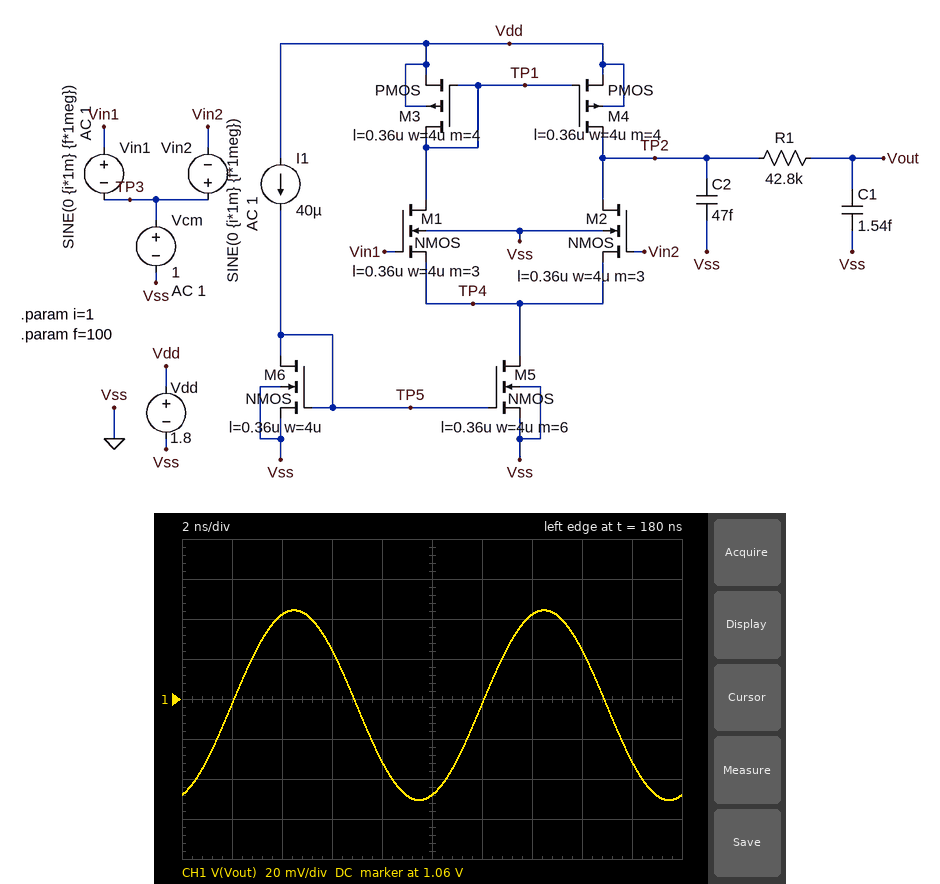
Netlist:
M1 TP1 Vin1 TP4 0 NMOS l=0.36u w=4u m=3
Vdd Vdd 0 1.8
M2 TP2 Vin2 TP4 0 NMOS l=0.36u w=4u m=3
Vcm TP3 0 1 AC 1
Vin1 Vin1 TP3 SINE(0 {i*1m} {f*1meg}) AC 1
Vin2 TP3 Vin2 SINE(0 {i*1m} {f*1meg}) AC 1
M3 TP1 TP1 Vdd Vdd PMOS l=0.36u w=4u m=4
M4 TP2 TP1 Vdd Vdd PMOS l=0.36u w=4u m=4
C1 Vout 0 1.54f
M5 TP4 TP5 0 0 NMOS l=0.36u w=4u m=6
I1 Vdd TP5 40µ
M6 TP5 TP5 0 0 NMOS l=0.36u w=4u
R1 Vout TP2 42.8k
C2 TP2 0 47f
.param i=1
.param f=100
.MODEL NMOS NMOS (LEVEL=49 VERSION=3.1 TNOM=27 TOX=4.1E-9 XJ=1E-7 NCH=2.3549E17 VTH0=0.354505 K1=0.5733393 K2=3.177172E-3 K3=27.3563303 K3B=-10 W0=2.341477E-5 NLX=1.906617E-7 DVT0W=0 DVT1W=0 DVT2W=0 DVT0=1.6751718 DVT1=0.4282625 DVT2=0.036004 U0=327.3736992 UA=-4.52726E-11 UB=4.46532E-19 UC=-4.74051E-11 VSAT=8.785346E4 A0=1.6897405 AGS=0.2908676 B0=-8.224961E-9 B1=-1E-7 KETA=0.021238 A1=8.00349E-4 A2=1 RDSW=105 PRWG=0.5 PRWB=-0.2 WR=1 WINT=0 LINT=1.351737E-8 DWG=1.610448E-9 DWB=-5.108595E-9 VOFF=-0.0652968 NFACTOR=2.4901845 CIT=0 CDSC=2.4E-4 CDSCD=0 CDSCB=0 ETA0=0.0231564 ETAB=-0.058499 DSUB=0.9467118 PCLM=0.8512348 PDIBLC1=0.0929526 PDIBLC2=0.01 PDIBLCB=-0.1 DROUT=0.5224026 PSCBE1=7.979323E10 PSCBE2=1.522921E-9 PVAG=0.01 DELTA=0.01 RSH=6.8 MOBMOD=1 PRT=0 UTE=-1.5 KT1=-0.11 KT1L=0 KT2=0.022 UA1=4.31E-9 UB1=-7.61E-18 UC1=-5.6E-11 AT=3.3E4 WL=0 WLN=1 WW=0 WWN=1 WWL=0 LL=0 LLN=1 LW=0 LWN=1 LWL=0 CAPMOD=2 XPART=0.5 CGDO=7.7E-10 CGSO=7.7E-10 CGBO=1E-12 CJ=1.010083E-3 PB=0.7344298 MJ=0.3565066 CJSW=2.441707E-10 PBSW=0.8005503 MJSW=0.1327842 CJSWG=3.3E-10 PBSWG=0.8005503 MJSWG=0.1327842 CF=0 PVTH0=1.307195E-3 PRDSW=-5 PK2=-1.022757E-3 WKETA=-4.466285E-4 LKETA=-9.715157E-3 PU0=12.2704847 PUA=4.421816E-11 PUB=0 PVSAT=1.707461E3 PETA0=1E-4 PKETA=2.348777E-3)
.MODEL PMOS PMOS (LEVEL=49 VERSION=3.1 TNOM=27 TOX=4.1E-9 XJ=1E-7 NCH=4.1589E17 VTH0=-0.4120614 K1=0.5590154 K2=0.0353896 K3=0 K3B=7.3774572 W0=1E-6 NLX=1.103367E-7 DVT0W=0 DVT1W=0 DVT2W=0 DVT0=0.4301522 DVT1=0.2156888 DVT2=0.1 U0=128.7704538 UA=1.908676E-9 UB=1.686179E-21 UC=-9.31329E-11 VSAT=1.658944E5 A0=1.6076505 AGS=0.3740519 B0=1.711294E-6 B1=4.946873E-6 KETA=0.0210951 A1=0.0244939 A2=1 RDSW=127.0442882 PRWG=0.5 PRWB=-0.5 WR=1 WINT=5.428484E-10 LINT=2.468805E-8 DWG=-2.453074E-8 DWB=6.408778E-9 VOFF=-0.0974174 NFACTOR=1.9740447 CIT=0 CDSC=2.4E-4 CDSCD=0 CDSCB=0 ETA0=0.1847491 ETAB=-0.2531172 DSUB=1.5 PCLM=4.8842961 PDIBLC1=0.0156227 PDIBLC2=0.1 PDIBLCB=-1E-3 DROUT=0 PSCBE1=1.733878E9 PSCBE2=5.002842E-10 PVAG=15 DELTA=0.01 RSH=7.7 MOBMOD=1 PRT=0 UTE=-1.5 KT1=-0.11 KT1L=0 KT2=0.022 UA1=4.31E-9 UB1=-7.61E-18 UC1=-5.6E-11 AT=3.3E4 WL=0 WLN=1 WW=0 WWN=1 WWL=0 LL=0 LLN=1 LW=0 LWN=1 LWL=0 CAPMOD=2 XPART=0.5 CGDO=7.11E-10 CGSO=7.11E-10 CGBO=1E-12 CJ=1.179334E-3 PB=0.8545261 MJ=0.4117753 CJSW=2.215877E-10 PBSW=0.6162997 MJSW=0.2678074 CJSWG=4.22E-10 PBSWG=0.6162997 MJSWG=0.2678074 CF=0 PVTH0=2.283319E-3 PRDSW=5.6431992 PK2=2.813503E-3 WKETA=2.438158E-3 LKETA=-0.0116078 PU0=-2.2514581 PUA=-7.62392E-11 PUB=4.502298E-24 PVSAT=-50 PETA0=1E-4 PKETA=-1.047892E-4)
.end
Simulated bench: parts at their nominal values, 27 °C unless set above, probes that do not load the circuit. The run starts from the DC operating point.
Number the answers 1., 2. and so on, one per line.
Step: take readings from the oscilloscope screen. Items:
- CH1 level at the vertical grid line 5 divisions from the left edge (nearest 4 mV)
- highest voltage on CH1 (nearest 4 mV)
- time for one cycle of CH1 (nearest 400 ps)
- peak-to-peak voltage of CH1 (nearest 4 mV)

1. 1.012 V
2. 1.104 V
3. 10.0 ns
4. 96 mV
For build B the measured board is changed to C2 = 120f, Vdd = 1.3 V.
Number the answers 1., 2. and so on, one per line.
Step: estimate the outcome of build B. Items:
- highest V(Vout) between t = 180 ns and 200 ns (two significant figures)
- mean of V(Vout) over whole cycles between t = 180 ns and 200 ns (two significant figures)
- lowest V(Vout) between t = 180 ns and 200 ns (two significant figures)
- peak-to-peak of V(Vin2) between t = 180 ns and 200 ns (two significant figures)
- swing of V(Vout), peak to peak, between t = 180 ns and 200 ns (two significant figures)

1. 580 mV
2. 560 mV
3. 530 mV
4. 2.0 mV
5. 50 mV
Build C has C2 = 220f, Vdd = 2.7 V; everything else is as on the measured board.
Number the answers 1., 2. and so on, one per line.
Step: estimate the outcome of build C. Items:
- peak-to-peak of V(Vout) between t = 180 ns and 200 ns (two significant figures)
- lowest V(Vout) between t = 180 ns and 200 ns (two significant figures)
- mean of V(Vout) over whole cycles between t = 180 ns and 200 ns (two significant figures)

1. 34 mV
2. 1.9 V
3. 2.0 V
